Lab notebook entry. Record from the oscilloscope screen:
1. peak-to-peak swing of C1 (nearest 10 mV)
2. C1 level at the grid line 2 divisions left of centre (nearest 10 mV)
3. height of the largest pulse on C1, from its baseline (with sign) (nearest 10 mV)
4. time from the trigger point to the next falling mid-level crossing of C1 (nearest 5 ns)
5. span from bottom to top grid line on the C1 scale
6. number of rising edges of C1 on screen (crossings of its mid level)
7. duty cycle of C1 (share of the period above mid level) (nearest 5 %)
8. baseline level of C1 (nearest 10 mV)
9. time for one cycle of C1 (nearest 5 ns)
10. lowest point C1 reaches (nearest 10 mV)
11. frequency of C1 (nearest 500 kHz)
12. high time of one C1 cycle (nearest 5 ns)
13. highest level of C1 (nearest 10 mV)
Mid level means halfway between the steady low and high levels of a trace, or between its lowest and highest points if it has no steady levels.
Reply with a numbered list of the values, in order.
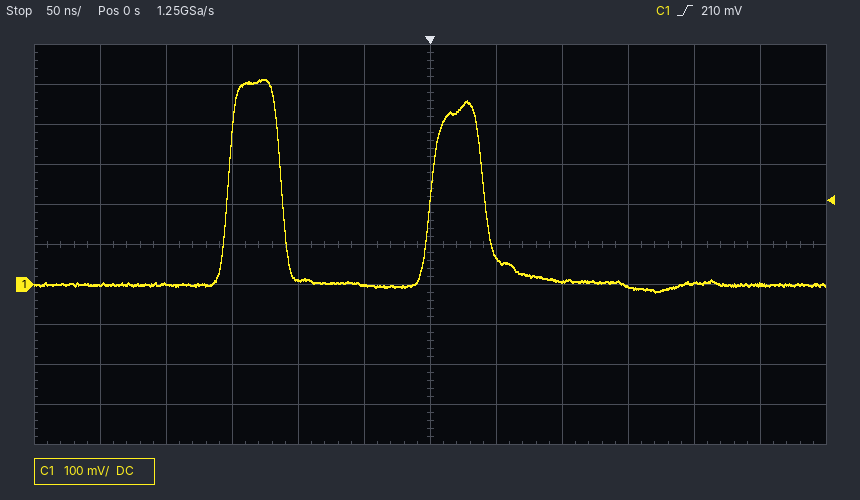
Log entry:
1. 530 mV
2. 10 mV
3. +510 mV
4. 40 ns
5. 1 V
6. 2
7. 25 %
8. 0 mV
9. 155 ns
10. -20 mV
11. 6.5 MHz
12. 40 ns
13. 510 mV
